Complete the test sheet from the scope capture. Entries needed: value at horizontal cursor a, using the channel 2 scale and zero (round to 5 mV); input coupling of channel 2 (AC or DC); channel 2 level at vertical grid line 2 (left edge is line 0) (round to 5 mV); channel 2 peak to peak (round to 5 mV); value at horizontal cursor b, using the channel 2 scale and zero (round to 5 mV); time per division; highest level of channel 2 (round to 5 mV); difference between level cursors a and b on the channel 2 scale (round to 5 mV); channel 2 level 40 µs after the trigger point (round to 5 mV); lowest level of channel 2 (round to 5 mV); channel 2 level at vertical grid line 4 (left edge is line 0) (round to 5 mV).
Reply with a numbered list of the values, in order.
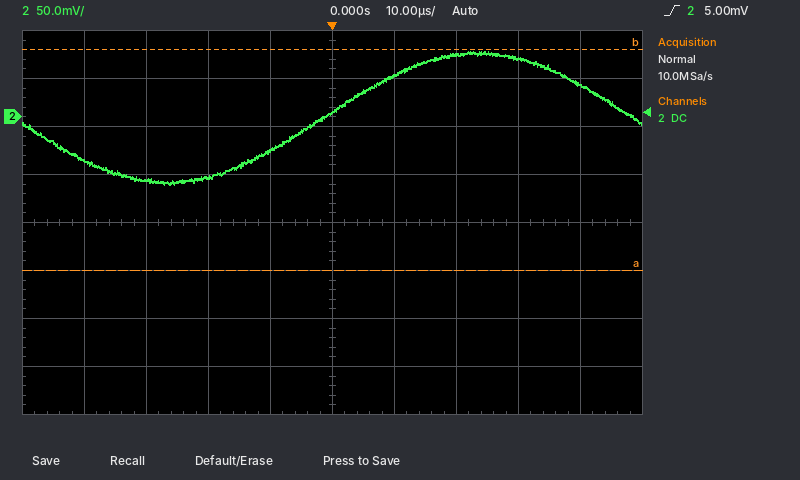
1. -160 mV
2. DC
3. -65 mV
4. 140 mV
5. 70 mV
6. 10 µs
7. 70 mV
8. 230 mV
9. 35 mV
10. -70 mV
11. -35 mV
